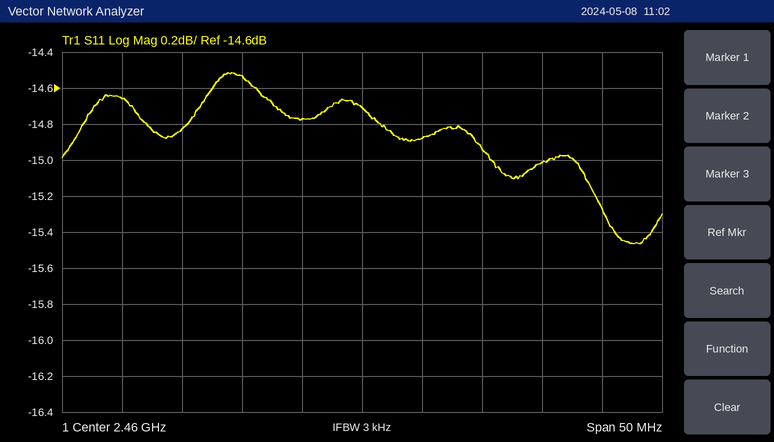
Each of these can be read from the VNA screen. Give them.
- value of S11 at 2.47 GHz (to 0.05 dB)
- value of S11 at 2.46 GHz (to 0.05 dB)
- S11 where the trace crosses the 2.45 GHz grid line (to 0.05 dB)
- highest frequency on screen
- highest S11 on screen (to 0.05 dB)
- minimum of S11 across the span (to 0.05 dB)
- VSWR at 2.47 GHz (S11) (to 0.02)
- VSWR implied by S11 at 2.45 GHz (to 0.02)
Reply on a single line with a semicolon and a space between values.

-14.95 dB; -14.70 dB; -14.55 dB; 2.485 GHz; -14.50 dB; -15.45 dB; 1.44; 1.46
